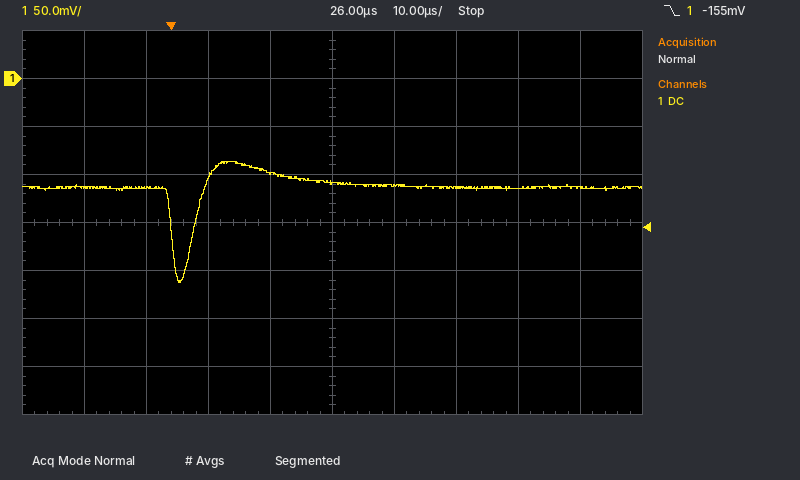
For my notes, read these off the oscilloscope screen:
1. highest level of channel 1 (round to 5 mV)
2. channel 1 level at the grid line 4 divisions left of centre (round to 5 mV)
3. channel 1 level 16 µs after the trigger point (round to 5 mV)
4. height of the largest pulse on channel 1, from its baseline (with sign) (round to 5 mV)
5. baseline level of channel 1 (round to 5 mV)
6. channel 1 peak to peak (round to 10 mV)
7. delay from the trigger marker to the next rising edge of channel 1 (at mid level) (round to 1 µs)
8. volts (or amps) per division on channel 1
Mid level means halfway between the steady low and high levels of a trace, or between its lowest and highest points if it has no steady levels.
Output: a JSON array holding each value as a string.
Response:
["-85 mV", "-115 mV", "-100 mV", "-100 mV", "-115 mV", "130 mV", "4 µs", "50 mV"]
